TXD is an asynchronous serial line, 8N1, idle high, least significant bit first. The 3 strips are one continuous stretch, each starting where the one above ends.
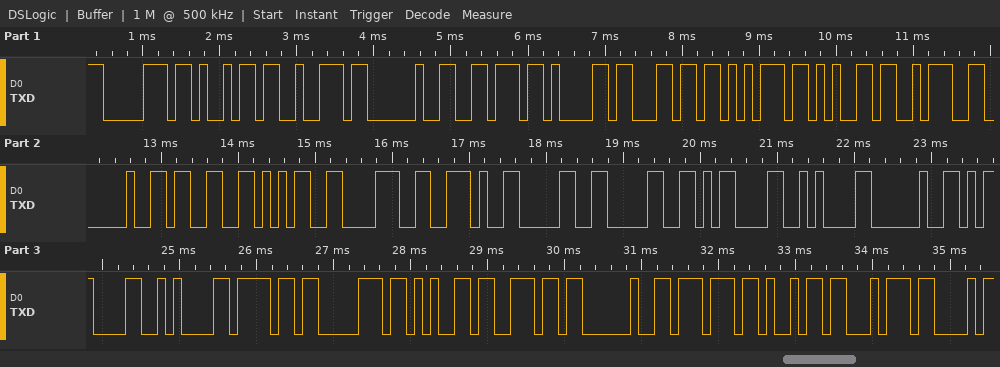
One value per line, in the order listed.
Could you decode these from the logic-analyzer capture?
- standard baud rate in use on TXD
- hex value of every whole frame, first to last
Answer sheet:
9600 baud
0x70 0x69 0x72 0x20 0x76 0x61 0x6C 0x75 0x65 0x3A 0x20 0x33 0x35 0x38 0x2E 0x30 0x30 0x0D 0x0A 0x20 0x0D 0x0A 0x6F 0x70 0x65 0x6E 0x20 0x77 0x69 0x74
